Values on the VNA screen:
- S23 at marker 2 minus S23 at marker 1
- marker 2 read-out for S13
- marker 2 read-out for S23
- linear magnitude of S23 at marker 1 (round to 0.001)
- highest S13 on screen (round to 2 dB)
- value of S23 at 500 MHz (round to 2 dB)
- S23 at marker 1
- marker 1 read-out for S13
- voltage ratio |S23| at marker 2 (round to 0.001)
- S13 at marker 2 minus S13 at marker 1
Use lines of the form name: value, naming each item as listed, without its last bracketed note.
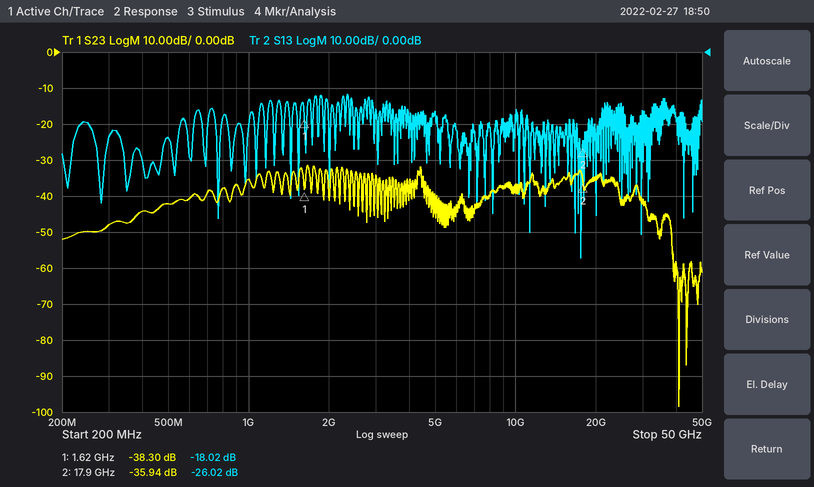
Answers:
S23 at marker 2 minus S23 at marker 1: 2.36 dB
marker 2 read-out for S13: -26.02 dB
marker 2 read-out for S23: -35.94 dB
linear magnitude of S23 at marker 1: 0.012
highest S13 on screen: -12 dB
value of S23 at 500 MHz: -42 dB
S23 at marker 1: -38.30 dB
marker 1 read-out for S13: -18.02 dB
voltage ratio |S23| at marker 2: 0.016
S13 at marker 2 minus S13 at marker 1: -8.00 dB
